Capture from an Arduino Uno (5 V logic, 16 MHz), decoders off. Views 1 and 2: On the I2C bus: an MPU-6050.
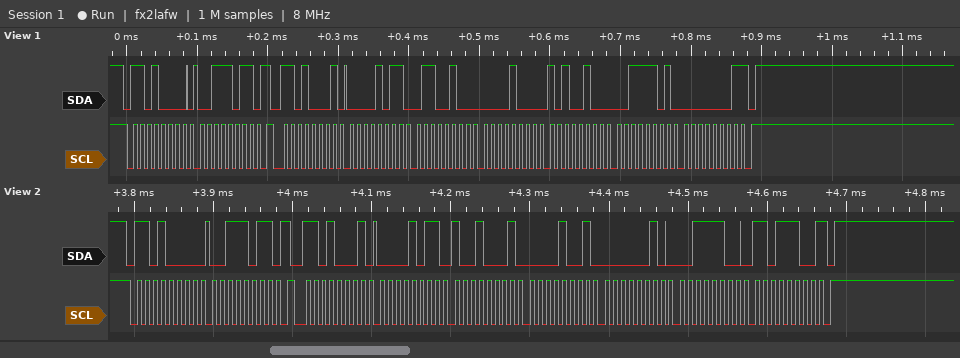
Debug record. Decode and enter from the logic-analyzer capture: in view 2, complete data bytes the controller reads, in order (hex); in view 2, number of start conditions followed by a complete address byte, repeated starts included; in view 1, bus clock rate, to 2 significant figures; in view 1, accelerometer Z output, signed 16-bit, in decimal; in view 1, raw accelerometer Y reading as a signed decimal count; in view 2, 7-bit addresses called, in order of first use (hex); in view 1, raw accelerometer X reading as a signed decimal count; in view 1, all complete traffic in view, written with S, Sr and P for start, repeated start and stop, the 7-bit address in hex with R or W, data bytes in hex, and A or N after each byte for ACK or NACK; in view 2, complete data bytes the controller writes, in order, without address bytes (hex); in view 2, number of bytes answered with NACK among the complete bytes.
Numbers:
0B 91 09 02 3C DC
2
100 kHz
15617
2212
0x68
2916
S 68W A 3B A Sr 68R A 0B A 64 A 08 A A4 A 3D A 01 N P
3B
1
